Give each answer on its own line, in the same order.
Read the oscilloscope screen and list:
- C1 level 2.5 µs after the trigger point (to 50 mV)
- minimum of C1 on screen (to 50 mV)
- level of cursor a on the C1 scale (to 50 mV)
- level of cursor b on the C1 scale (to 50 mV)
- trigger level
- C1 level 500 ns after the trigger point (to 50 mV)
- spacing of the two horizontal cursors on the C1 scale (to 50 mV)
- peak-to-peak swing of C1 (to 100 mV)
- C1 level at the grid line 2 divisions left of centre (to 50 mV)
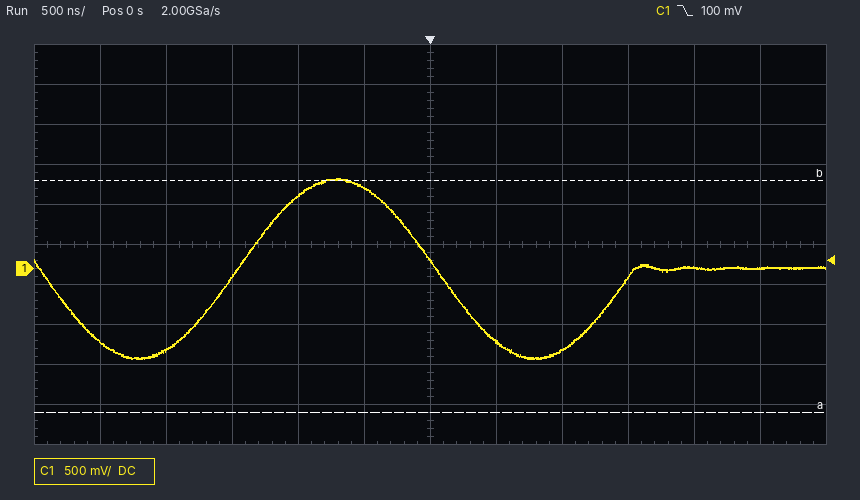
0 mV
-1.15 V
-1.80 V
1.10 V
100 mV
-900 mV
2.90 V
2.30 V
900 mV
